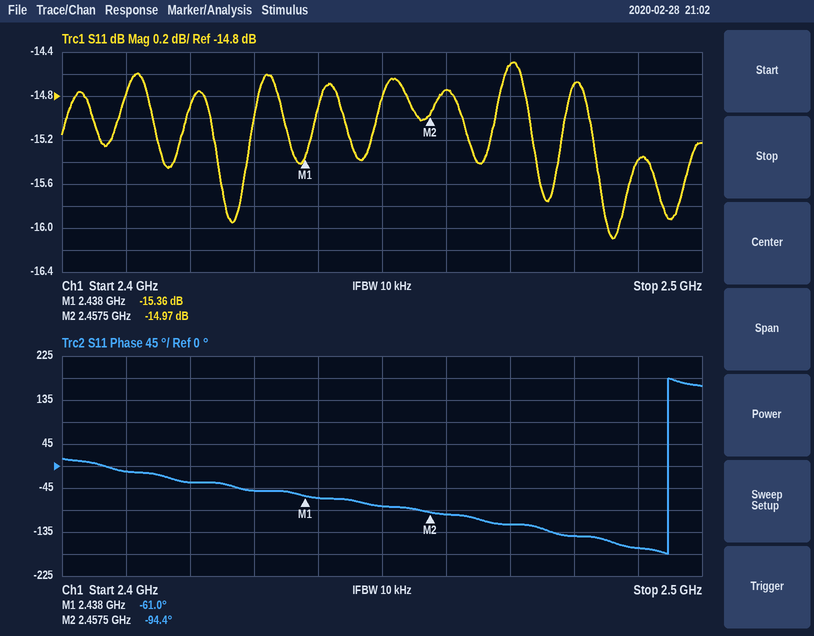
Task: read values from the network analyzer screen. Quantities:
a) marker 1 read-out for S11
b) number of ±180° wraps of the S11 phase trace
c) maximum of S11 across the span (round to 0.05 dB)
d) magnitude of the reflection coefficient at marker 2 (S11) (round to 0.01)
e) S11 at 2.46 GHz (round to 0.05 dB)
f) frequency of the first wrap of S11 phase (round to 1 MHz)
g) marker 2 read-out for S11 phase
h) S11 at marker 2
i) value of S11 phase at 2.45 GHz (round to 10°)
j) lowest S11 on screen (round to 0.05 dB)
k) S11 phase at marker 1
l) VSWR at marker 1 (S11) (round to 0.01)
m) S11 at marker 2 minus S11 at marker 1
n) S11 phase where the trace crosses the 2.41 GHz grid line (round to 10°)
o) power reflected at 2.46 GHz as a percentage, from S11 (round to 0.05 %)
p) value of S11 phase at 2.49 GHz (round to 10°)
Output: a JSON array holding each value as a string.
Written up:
["-15.36 dB", "1", "-14.50 dB", "0.18", "-14.75 dB", "2.495 GHz", "-94.4°", "-14.97 dB", "-80°", "-16.10 dB", "-61.0°", "1.41", "0.39 dB", "-10°", "3.35 %", "-170°"]
